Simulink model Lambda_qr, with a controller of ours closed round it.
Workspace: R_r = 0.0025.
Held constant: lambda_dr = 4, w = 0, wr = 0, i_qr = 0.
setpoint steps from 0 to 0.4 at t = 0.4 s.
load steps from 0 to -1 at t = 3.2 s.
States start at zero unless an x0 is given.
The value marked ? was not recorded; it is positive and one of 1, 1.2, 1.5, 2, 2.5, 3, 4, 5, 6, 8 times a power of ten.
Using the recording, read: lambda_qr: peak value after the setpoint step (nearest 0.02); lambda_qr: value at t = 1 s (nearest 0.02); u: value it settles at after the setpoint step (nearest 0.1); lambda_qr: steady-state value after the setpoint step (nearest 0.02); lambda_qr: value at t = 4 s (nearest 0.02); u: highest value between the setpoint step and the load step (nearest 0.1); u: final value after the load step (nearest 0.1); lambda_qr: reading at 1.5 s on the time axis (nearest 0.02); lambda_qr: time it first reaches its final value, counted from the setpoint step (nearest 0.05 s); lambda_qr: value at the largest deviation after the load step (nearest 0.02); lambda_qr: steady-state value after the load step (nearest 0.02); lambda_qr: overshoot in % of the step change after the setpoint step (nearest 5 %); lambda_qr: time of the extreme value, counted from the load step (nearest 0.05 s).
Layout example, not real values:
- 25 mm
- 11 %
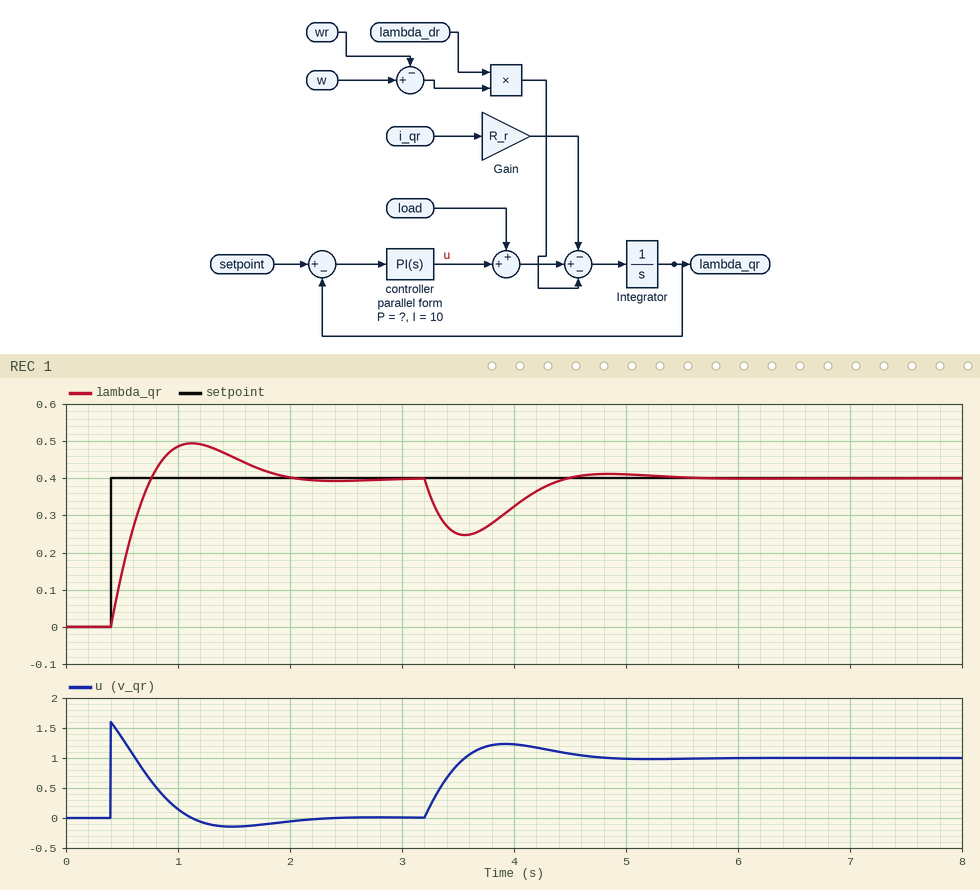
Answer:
- 0.50
- 0.48
- 0.0
- 0.40
- 0.32
- 1.6
- 1.0
- 0.46
- 0.35 s
- 0.24
- 0.40
- 25 %
- 0.35 s
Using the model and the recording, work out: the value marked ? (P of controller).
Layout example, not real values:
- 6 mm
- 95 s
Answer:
- 4
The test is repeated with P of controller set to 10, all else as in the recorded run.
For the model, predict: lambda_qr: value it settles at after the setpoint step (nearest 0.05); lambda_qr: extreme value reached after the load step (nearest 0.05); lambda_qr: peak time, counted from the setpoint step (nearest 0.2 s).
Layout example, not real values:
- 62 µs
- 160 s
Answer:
- 0.40
- 0.30
- 0.6 s
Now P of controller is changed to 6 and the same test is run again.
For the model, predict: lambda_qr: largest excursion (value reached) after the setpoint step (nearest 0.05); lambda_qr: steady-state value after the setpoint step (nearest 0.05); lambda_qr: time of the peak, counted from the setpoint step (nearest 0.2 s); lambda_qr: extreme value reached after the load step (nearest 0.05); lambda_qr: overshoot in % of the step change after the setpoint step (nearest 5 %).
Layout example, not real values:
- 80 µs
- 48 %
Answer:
- 0.45
- 0.40
- 0.6 s
- 0.30
- 15 %
